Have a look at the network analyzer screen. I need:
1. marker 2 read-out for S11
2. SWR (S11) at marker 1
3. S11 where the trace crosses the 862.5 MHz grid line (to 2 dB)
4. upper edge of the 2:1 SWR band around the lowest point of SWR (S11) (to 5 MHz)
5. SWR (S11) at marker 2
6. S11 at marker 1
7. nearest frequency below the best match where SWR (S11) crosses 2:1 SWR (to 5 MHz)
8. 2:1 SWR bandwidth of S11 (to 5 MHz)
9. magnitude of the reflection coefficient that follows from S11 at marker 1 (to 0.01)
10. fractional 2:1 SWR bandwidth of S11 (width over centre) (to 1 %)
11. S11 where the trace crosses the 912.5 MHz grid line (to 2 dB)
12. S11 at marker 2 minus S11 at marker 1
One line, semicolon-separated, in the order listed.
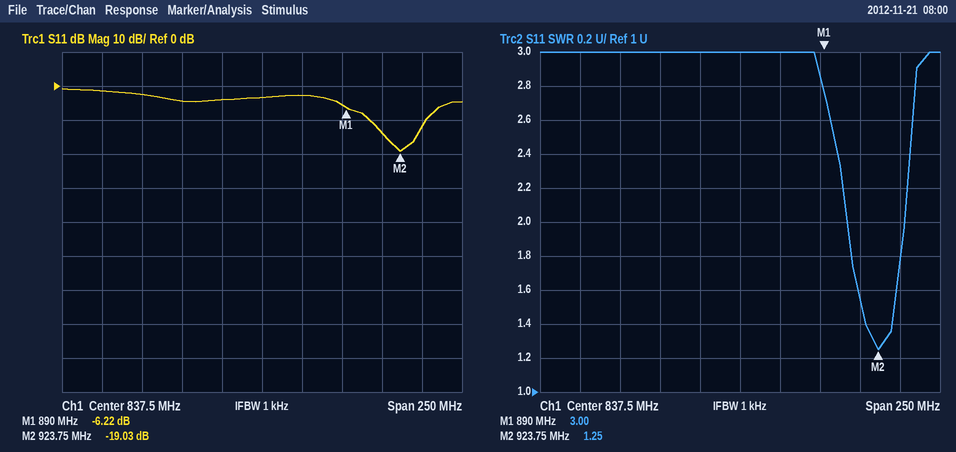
-19.03 dB; 3.00; -2 dB; 940 MHz; 1.25; -6.22 dB; 905 MHz; 35 MHz; 0.49; 4 %; -14 dB; -12.81 dB
